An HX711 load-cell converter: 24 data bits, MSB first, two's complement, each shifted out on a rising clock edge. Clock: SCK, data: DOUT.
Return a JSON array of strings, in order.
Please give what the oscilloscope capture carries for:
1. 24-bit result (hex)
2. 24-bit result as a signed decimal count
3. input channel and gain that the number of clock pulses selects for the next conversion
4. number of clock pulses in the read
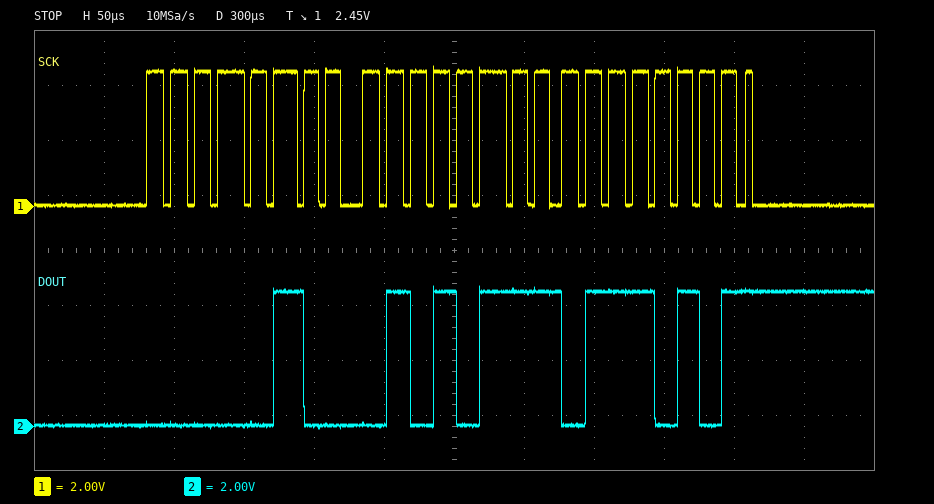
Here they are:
["0x045775", "284533", "channel A, gain 128", "25"]
